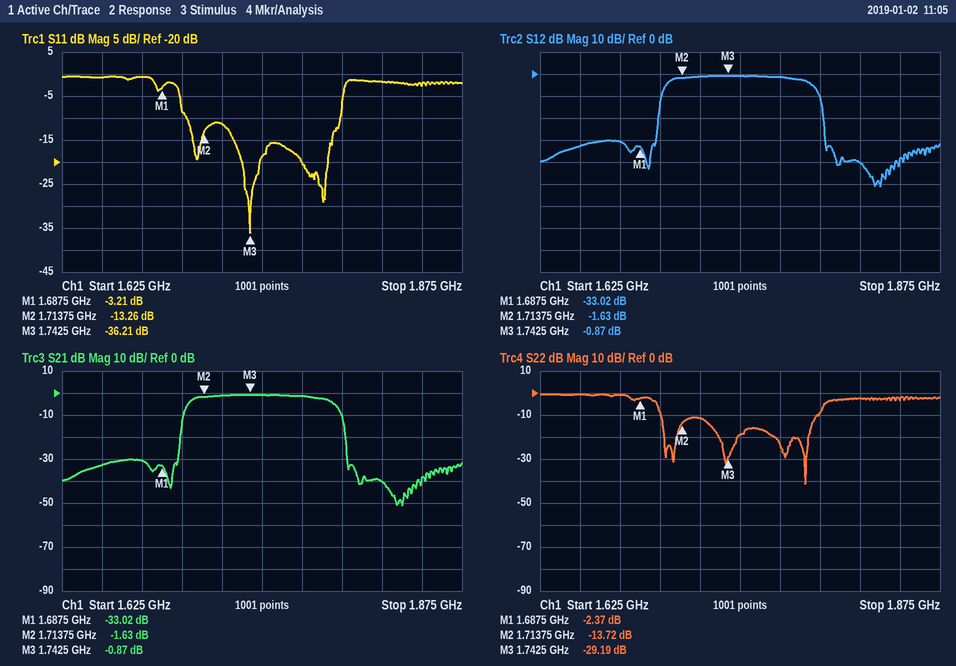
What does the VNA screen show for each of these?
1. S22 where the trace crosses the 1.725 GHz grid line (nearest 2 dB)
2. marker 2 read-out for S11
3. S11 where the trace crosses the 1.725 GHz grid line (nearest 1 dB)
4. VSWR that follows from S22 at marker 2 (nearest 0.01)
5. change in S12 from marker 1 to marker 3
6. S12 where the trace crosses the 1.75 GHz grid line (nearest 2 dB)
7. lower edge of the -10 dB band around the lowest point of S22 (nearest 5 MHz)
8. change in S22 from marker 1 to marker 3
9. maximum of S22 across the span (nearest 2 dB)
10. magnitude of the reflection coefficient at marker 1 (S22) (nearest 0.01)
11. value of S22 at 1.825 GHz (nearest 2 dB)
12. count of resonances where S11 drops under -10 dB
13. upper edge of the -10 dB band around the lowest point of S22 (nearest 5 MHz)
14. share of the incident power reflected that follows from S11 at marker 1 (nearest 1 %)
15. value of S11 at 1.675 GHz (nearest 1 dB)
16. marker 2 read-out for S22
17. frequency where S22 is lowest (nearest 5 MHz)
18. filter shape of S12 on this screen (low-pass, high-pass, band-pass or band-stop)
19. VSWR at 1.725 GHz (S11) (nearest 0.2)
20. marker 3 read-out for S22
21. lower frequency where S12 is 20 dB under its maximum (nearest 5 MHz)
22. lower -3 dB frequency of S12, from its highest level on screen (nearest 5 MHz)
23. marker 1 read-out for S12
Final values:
-12 dB
-13.26 dB
-11 dB
1.52
32.15 dB
0 dB
1.700 GHz
-26.82 dB
0 dB
0.76
-2 dB
3
1.800 GHz
48 %
-1 dB
-13.72 dB
1.790 GHz
band-pass
1.8
-29.19 dB
1.700 GHz
1.705 GHz
-33.02 dB
